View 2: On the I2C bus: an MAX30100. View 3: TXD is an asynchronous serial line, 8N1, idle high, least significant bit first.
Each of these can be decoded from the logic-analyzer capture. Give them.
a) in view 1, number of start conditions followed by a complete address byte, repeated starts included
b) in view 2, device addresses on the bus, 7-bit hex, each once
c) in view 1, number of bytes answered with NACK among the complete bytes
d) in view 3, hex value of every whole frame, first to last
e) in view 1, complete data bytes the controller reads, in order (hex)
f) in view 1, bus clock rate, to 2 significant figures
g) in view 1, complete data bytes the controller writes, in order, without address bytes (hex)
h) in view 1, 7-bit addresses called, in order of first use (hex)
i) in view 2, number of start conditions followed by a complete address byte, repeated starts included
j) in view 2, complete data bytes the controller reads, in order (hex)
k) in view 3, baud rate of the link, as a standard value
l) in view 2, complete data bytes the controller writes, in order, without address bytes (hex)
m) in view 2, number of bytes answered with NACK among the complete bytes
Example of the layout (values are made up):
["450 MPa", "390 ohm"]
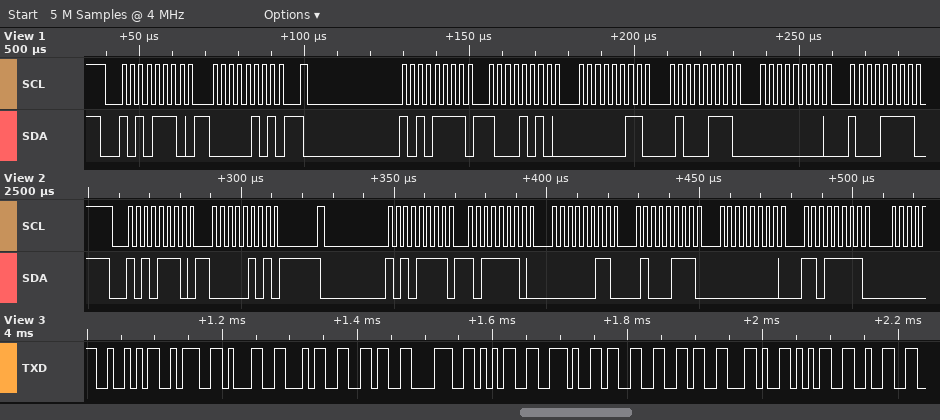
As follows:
["2", "0x57", "0", "52 3A 31 34 36 38 35 2E 33 36 2C 35 32", "8A 03 47 00 8F", "400 kHz", "05", "0x57", "2", "BE 03 47 00 DF", "115200 baud", "05", "0"]
